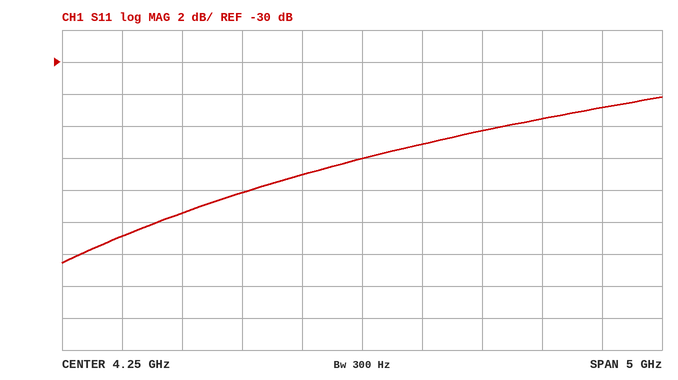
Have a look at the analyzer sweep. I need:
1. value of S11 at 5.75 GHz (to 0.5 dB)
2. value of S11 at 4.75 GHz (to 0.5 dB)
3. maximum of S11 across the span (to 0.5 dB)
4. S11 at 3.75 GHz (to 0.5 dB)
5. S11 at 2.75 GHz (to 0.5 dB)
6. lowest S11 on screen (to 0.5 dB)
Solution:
-33.5 dB
-35.0 dB
-32.0 dB
-37.0 dB
-39.5 dB
-42.5 dB
